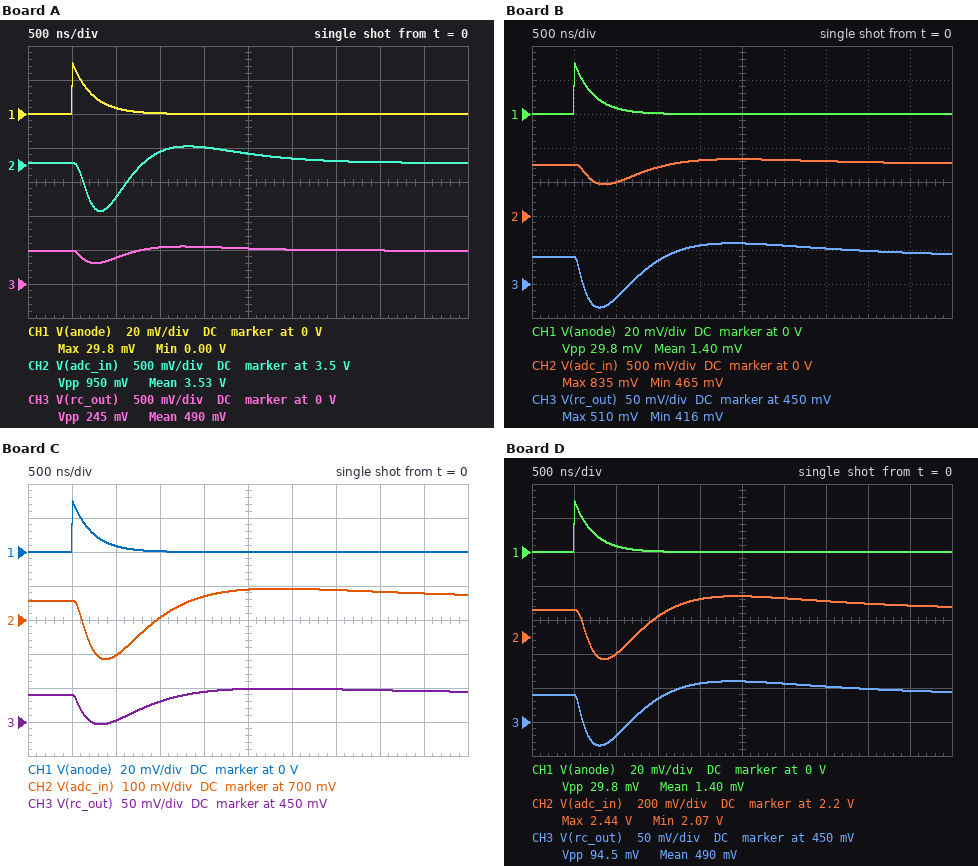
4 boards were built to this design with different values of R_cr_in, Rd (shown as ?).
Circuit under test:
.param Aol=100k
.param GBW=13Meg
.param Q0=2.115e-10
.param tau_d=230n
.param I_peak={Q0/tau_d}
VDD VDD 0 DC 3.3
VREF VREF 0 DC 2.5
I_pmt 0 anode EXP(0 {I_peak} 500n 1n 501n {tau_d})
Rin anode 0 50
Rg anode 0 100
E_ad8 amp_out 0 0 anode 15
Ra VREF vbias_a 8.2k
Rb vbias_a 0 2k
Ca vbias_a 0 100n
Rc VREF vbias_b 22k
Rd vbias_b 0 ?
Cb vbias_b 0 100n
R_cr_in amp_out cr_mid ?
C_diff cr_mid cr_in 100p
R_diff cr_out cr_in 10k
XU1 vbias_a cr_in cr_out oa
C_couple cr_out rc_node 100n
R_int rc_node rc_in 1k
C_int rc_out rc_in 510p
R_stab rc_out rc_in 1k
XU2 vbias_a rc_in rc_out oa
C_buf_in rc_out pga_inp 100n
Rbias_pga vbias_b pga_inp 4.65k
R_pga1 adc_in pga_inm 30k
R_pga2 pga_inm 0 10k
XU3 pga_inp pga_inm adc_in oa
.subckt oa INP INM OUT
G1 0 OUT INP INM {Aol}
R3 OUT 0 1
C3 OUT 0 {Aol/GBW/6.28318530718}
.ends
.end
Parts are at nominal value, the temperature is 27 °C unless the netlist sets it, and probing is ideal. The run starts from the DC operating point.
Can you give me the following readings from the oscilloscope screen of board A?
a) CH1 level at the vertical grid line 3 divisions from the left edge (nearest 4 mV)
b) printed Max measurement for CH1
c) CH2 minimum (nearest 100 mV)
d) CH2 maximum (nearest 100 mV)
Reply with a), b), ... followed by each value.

a) 0 V
b) 29.8 mV
c) 2.8 V
d) 3.8 V
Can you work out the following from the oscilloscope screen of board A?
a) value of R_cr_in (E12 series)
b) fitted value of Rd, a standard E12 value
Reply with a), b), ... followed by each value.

a) 3.9 kΩ
b) 12 kΩ
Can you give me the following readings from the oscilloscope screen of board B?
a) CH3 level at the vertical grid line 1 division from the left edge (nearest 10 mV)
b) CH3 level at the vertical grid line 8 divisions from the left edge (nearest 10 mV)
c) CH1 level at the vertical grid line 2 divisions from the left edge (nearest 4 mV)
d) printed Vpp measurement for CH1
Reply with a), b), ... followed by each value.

a) 490 mV
b) 500 mV
c) 4 mV
d) 29.8 mV
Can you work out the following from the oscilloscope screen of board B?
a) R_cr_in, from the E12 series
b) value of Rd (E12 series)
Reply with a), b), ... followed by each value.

a) 12 kΩ
b) 1.8 kΩ
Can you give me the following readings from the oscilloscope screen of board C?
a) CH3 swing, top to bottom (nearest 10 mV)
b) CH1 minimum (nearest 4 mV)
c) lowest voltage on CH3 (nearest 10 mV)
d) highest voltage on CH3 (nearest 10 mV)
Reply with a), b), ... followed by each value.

a) 50 mV
b) 0 V
c) 450 mV
d) 500 mV
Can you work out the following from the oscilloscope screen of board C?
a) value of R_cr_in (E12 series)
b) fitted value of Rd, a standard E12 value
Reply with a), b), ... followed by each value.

a) 22 kΩ
b) 1.8 kΩ
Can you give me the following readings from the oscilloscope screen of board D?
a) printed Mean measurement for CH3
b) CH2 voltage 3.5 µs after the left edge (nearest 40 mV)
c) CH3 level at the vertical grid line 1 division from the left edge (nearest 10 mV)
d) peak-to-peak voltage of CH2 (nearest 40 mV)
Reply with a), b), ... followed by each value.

a) 490 mV
b) 2.40 V
c) 490 mV
d) 360 mV
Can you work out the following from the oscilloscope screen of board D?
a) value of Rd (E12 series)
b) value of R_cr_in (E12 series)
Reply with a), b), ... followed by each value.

a) 6.8 kΩ
b) 12 kΩ
